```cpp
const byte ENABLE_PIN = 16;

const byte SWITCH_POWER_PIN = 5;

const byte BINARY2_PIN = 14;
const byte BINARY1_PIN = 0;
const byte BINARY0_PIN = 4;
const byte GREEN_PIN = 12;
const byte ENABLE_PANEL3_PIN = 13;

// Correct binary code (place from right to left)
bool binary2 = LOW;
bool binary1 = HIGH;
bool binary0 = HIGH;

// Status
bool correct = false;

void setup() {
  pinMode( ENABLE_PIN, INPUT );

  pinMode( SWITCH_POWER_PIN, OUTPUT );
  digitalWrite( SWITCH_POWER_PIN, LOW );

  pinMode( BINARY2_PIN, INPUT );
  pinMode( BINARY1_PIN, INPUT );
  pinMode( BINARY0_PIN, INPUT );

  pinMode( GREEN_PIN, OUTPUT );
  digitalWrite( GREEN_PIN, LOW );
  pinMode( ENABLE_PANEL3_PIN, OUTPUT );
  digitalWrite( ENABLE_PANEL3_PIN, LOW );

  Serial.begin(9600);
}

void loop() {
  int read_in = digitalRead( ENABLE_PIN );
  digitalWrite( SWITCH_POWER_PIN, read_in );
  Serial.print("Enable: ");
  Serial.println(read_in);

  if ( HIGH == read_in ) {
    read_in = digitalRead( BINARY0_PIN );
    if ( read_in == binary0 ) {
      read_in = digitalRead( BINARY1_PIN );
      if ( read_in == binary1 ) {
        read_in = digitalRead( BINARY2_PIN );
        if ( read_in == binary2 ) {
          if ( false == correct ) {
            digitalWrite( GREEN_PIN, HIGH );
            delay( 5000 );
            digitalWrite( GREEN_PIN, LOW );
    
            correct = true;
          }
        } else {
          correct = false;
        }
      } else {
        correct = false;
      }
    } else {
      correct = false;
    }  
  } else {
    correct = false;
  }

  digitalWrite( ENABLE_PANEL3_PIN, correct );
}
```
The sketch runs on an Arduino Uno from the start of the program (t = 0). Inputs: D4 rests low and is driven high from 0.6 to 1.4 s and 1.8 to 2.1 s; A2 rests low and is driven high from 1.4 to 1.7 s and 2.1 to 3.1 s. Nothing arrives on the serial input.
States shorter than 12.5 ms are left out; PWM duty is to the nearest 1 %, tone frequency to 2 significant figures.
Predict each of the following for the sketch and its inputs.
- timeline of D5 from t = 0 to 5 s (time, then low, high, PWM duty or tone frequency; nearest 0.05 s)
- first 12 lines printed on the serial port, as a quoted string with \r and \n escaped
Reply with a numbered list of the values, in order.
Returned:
1. 0 s low; 1.4 s high; 1.7 s low; 2.1 s high; 3.1 s low
2. "Enable: 0\r\nEnable: 0\r\nEnable: 0\r\nEnable: 0\r\nEnable: 0\r\nEnable: 0\r\nEnable: 0\r\nEnable: 0\r\nEnable: 0\r\nEnable: 0\r\nEnable: 0\r\nEnable: 0\r\n"
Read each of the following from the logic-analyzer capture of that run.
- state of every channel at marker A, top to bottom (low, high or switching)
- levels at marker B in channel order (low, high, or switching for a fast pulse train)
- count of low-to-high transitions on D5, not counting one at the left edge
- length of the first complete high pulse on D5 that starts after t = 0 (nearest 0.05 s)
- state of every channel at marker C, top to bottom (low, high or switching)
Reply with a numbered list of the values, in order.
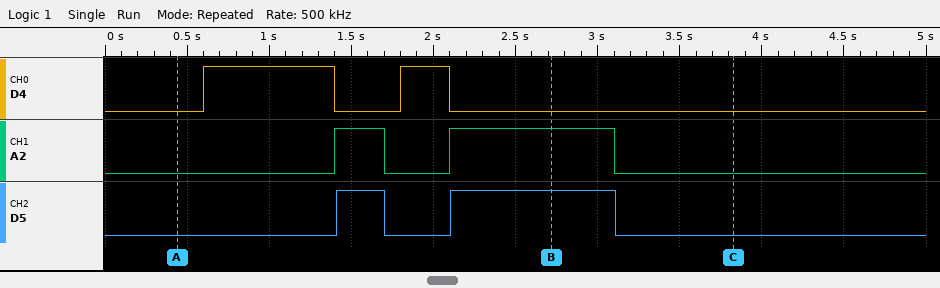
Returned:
1. D4 low, A2 low, D5 low
2. D4 low, A2 high, D5 high
3. 2
4. 0.30 s
5. D4 low, A2 low, D5 low
